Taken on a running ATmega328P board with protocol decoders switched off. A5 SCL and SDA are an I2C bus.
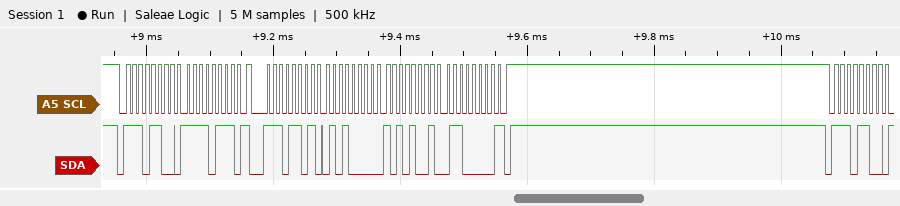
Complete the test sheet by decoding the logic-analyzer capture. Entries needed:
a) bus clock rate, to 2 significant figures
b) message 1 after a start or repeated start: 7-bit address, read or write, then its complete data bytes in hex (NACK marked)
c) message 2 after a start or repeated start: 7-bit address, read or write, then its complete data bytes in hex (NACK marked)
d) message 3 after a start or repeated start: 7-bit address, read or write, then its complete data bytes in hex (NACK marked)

100 kHz
0x76 write: F7
0x76 read: 50 A9 60 NACK
0x76 write
